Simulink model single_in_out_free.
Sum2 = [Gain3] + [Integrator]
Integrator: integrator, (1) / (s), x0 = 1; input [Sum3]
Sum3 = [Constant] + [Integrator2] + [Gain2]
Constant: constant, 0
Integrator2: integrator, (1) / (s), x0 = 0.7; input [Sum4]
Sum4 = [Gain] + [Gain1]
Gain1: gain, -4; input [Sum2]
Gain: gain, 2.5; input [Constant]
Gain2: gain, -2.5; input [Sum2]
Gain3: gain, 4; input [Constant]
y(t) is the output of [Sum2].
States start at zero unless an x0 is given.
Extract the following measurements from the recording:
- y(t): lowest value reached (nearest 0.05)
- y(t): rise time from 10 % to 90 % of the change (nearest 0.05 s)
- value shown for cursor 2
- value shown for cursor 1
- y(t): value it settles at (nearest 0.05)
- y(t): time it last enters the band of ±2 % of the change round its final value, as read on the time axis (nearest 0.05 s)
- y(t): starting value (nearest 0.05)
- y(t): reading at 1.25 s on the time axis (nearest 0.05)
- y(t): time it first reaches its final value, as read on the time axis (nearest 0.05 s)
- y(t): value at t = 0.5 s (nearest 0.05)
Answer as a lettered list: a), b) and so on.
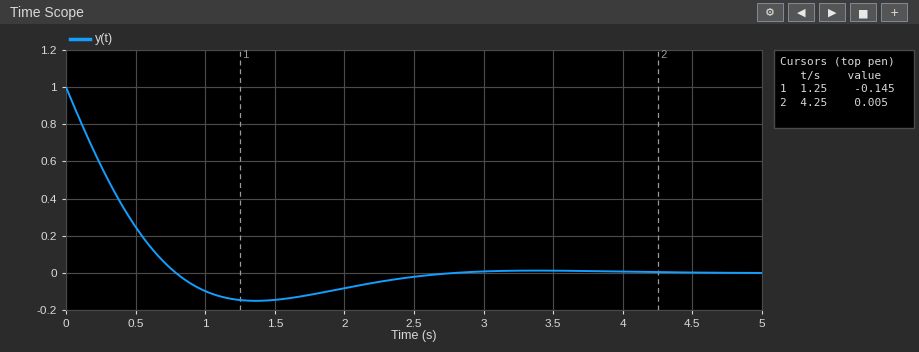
a) -0.15
b) 0.60 s
c) 0.005
d) -0.145
e) 0.00
f) 2.50 s
g) 1.00
h) -0.15
i) 0.80 s
j) 0.25
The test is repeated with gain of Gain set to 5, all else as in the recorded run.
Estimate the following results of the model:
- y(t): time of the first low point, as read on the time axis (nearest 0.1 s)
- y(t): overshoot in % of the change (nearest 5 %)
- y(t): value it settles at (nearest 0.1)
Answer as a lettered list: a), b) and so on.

a) 1.4 s
b) 15 %
c) 0.0
